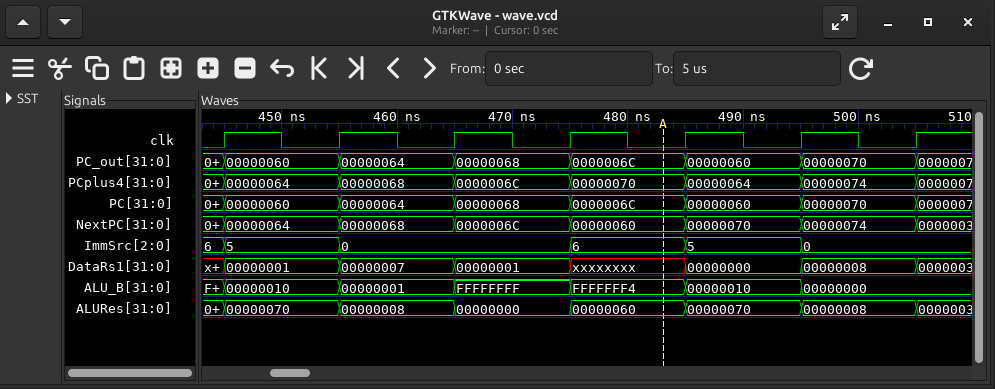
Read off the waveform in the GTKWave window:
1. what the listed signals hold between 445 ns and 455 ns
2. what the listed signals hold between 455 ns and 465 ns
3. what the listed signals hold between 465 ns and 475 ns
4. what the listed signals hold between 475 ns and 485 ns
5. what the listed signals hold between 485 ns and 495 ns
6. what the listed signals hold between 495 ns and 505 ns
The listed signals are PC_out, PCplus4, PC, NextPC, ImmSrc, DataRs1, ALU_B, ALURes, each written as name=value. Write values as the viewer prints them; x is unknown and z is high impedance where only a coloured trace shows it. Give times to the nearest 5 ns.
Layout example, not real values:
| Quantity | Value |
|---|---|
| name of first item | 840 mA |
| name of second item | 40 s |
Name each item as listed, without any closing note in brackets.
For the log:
| Quantity | Value |
|---|---|
| what the listed signals hold between 445 ns and 455 ns | PC_out=00000060, PCplus4=00000064, PC=00000060, NextPC=00000064, ImmSrc=5, DataRs1=00000001, ALU_B=00000010, ALURes=00000070 |
| what the listed signals hold between 455 ns and 465 ns | PC_out=00000064, PCplus4=00000068, PC=00000064, NextPC=00000068, ImmSrc=0, DataRs1=00000007, ALU_B=00000001, ALURes=00000008 |
| what the listed signals hold between 465 ns and 475 ns | PC_out=00000068, PCplus4=0000006C, PC=00000068, NextPC=0000006C, ImmSrc=0, DataRs1=00000001, ALU_B=FFFFFFFF, ALURes=00000000 |
| what the listed signals hold between 475 ns and 485 ns | PC_out=0000006C, PCplus4=00000070, PC=0000006C, NextPC=00000060, ImmSrc=6, DataRs1=xxxxxxxx, ALU_B=FFFFFFF4, ALURes=00000060 |
| what the listed signals hold between 485 ns and 495 ns | PC_out=00000060, PCplus4=00000064, PC=00000060, NextPC=00000070, ImmSrc=5, DataRs1=00000000, ALU_B=00000010, ALURes=00000070 |
| what the listed signals hold between 495 ns and 505 ns | PC_out=00000070, PCplus4=00000074, PC=00000070, NextPC=00000074, ImmSrc=0, DataRs1=00000008, ALU_B=00000000, ALURes=00000008 |
